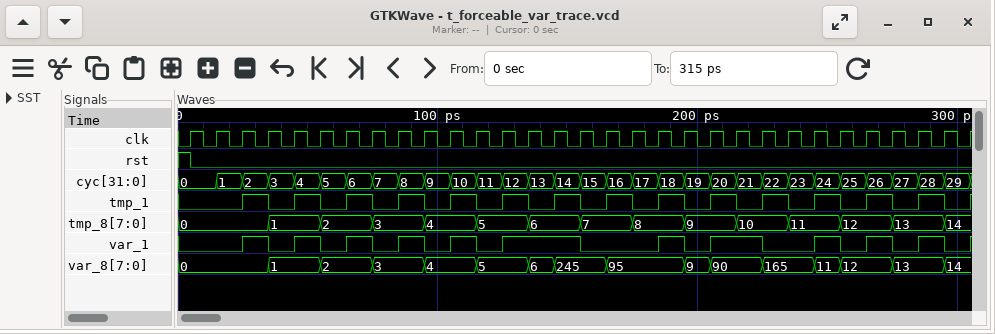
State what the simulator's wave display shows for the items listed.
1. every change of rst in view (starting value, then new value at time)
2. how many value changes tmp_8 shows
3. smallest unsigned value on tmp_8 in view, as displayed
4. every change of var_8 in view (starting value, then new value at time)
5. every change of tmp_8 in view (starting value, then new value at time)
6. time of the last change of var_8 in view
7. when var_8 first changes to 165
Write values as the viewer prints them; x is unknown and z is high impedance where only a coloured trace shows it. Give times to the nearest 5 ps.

1, 0 at 5 ps
14
0
0, 1 at 35 ps, 2 at 55 ps, 3 at 75 ps, 4 at 95 ps, 5 at 115 ps, 6 at 135 ps, 245 at 145 ps, 95 at 165 ps, 9 at 195 ps, 90 at 205 ps, 165 at 225 ps, 11 at 245 ps, 12 at 255 ps, 13 at 275 ps, 14 at 295 ps
0, 1 at 35 ps, 2 at 55 ps, 3 at 75 ps, 4 at 95 ps, 5 at 115 ps, 6 at 135 ps, 7 at 155 ps, 8 at 175 ps, 9 at 195 ps, 10 at 215 ps, 11 at 235 ps, 12 at 255 ps, 13 at 275 ps, 14 at 295 ps
295 ps
225 ps
